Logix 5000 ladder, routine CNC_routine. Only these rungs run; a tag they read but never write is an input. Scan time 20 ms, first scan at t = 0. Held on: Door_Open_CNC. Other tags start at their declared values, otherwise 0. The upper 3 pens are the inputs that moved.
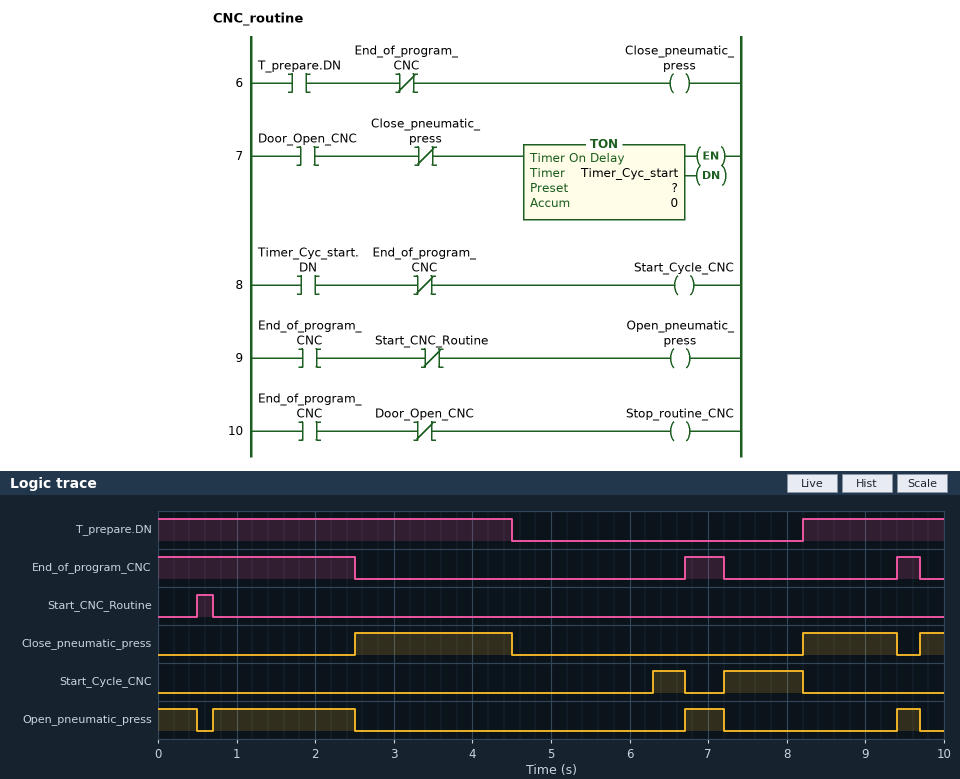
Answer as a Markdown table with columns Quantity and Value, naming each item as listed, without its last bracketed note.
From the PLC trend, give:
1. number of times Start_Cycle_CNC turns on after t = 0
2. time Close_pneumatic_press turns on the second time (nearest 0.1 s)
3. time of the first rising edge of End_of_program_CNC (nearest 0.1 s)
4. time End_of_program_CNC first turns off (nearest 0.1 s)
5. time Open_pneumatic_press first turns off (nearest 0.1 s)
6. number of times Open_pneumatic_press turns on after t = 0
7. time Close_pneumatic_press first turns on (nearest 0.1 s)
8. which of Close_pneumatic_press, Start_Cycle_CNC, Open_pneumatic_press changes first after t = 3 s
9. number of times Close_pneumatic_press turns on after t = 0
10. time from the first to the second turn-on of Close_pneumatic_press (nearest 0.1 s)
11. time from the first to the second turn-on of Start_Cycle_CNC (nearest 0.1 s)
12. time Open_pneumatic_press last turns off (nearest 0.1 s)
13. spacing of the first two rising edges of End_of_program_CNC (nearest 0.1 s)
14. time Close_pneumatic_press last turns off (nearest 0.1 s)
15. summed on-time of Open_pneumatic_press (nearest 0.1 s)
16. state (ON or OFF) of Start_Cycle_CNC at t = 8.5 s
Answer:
| Quantity | Value |
|---|---|
| number of times Start_Cycle_CNC turns on after t = 0 | 2 |
| time Close_pneumatic_press turns on the second time | 8.2 s |
| time of the first rising edge of End_of_program_CNC | 6.7 s |
| time End_of_program_CNC first turns off | 2.5 s |
| time Open_pneumatic_press first turns off | 0.5 s |
| number of times Open_pneumatic_press turns on after t = 0 | 3 |
| time Close_pneumatic_press first turns on | 2.5 s |
| which of Close_pneumatic_press, Start_Cycle_CNC, Open_pneumatic_press changes first after t = 3 s | Close_pneumatic_press |
| number of times Close_pneumatic_press turns on after t = 0 | 3 |
| time from the first to the second turn-on of Close_pneumatic_press | 5.7 s |
| time from the first to the second turn-on of Start_Cycle_CNC | 0.9 s |
| time Open_pneumatic_press last turns off | 9.7 s |
| spacing of the first two rising edges of End_of_program_CNC | 2.7 s |
| time Close_pneumatic_press last turns off | 9.4 s |
| summed on-time of Open_pneumatic_press | 3.1 s |
| state (ON or OFF) of Start_Cycle_CNC at t = 8.5 s | OFF |
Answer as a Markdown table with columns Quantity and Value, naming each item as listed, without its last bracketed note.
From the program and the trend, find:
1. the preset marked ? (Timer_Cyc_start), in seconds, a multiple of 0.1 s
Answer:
| Quantity | Value |
|---|---|
| the preset marked ? (Timer_Cyc_start), in seconds, a multiple of 0.1 s | 1.8 s |
